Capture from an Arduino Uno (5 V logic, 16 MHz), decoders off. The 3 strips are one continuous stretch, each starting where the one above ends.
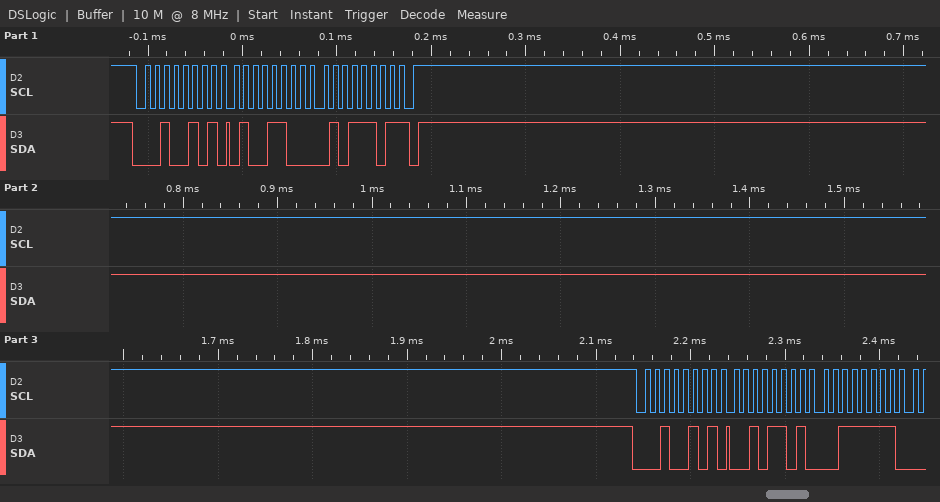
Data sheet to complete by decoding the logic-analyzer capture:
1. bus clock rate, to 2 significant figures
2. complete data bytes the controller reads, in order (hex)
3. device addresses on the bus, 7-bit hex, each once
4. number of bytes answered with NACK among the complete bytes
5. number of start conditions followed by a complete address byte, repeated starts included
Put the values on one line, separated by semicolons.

100 kHz; 4C 5D 2D 3F; 0x12; 1; 2
